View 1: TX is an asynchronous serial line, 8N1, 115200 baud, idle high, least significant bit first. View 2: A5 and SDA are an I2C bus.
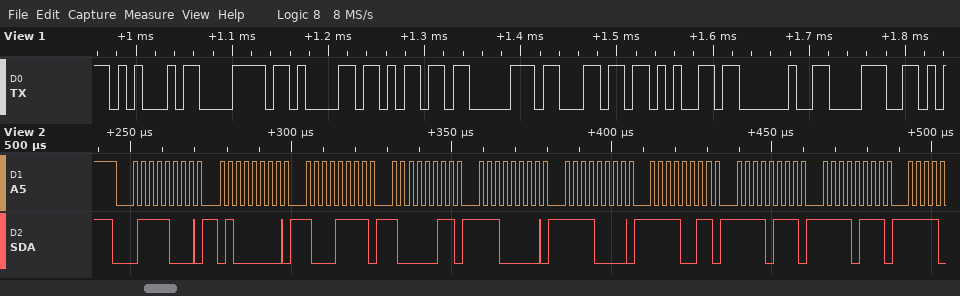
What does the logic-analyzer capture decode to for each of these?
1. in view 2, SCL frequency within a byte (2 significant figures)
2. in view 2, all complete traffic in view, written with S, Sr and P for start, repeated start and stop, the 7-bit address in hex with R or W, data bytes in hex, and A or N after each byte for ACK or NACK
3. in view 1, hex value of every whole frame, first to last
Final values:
400 kHz
S 3CW A 40 A 8F A 83 A E0 A F0 A F3 A F7 A F7 A
45 78 61 6D 70 6C 65 20 38
